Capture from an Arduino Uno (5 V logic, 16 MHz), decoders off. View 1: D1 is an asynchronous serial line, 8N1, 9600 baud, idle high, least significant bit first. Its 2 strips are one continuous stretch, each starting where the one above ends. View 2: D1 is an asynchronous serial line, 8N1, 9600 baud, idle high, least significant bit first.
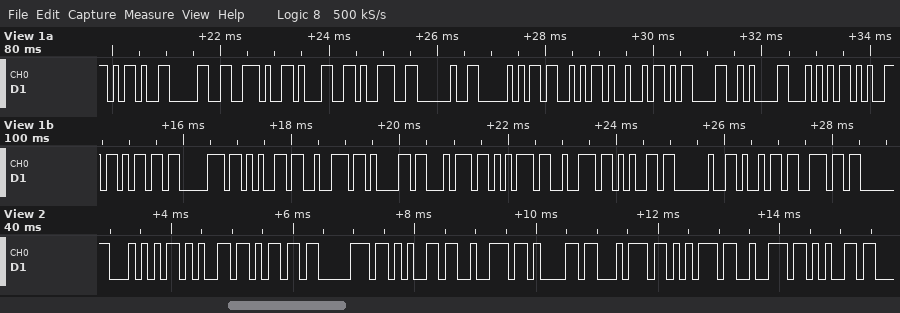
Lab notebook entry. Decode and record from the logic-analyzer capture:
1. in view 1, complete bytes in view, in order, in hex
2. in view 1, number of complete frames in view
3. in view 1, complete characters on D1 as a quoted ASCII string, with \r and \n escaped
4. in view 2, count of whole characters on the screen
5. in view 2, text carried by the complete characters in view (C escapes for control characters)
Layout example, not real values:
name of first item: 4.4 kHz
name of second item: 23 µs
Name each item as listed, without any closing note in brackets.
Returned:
in view 1, complete bytes in view, in order, in hex: 0x2D 0x30 0x2E 0x31 0x39 0x20 0x50 0x53 0x49 0x0D 0x0A 0x54 0x65 0x6D 0x70 0x65 0x72 0x61 0x74 0x75 0x72 0x65 0x20 0x69 0x6E
in view 1, number of complete frames in view: 25
in view 1, complete characters on D1 as a quoted ASCII string, with \r and \n escaped: "-0.19 PSI\r\nTemperature in"
in view 2, count of whole characters on the screen: 11
in view 2, text carried by the complete characters in view: "Temperature"
